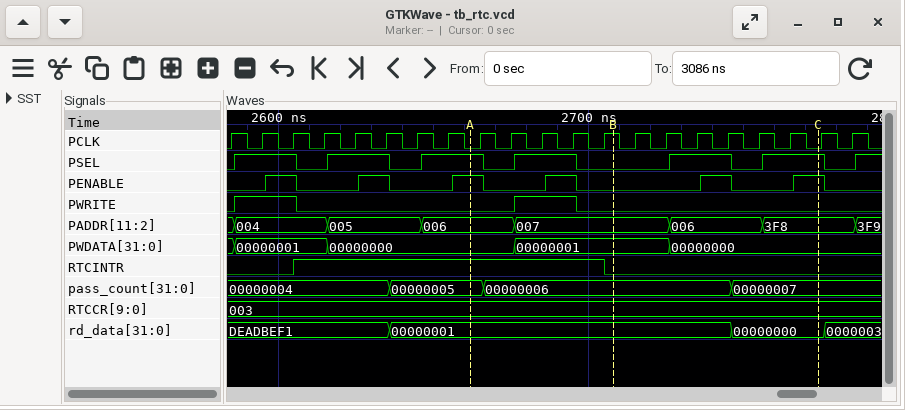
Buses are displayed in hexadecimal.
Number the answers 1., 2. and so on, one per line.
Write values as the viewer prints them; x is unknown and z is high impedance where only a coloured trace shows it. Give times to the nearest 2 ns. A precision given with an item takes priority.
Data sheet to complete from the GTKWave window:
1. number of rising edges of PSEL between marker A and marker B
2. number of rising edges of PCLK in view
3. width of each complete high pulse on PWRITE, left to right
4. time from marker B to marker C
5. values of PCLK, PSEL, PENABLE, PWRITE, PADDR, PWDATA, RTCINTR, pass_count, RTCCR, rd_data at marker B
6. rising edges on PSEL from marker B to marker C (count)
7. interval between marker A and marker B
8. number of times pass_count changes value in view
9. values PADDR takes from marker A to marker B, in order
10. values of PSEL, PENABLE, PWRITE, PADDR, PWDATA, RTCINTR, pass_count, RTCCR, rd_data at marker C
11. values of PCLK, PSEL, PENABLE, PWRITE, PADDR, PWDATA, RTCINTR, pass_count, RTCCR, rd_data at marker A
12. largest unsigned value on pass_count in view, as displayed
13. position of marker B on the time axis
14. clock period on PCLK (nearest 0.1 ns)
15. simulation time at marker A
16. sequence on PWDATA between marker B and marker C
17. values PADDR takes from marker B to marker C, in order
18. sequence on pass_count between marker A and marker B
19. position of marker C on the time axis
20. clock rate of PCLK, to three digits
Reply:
1. 1
2. 21
3. 20 ns, 20 ns
4. 66 ns
5. PCLK=1, PSEL=0, PENABLE=0, PWRITE=0, PADDR=007, PWDATA=00000001, RTCINTR=0, pass_count=00000006, RTCCR=003, rd_data=00000001
6. 2
7. 46 ns
8. 3
9. 006, 007
10. PSEL=1, PENABLE=1, PWRITE=0, PADDR=3F8, PWDATA=00000000, RTCINTR=0, pass_count=00000007, RTCCR=003, rd_data=00000000
11. PCLK=0, PSEL=1, PENABLE=1, PWRITE=0, PADDR=006, PWDATA=00000000, RTCINTR=1, pass_count=00000005, RTCCR=003, rd_data=00000001
12. 00000007
13. 2708 ns
14. 10 ns
15. 2662 ns
16. 00000001, 00000000
17. 007, 006, 3F8
18. 00000005, 00000006
19. 2774 ns
20. 100 MHz
